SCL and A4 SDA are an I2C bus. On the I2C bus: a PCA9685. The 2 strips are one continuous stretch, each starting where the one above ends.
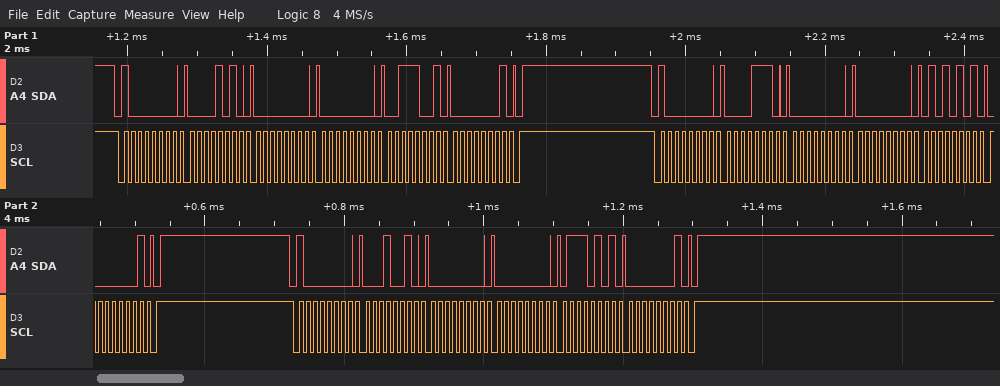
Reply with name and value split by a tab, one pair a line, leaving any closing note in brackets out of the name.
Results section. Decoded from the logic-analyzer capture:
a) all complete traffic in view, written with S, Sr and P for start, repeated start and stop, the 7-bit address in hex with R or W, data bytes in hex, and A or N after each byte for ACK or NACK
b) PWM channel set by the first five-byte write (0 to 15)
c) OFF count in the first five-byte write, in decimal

all complete traffic in view, written with S, Sr and P for start, repeated start and stop, the 7-bit address in hex with R or W, data bytes in hex, and A or N after each byte for ACK or NACK	S 40W A 0A A 00 A 00 A 39 A 01 A P S 40W A 0E A 00 A 00 A 55 A 01 A P S 40W A 12 A 00 A 00 A 75 A 01 A P
PWM channel set by the first five-byte write	1
OFF count in the first five-byte write, in decimal	313
